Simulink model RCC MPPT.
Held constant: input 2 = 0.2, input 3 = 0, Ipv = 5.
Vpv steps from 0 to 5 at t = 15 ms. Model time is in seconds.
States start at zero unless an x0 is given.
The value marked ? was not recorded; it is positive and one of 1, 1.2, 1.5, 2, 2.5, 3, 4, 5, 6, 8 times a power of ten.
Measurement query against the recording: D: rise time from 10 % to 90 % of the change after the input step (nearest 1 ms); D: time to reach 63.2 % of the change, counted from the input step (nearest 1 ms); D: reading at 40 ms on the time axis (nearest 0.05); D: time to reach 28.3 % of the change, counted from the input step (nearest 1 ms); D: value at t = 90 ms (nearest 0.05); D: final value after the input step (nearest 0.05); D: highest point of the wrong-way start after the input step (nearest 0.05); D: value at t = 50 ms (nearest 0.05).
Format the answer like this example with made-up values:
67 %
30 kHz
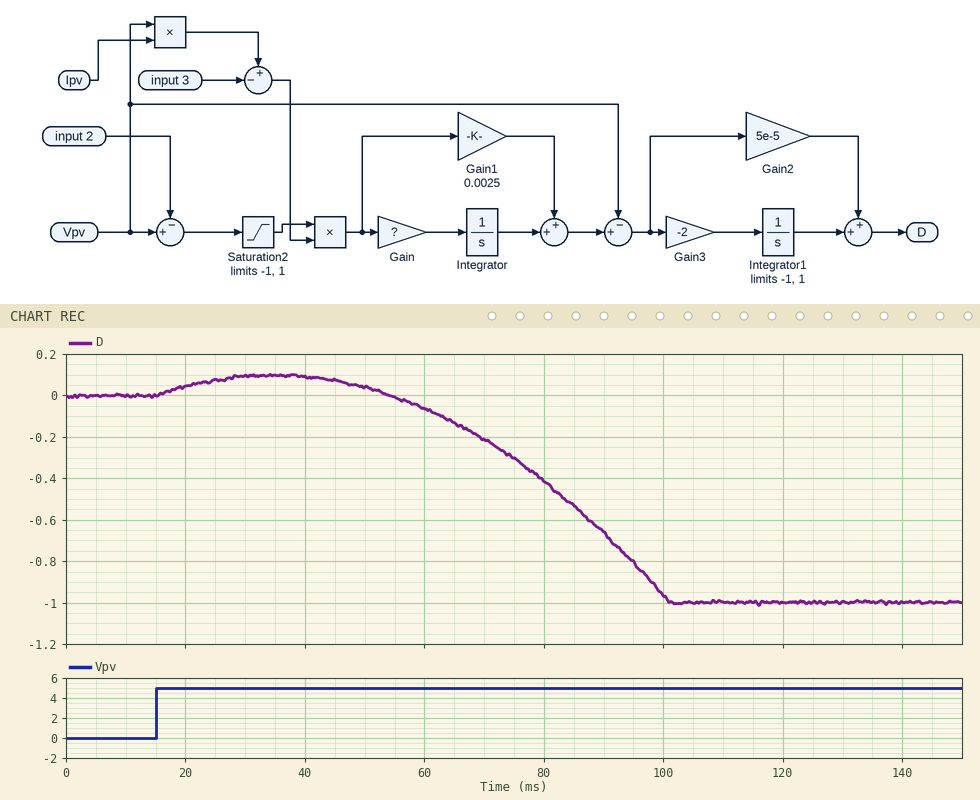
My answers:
35 ms
74 ms
0.10
59 ms
-0.65
-1.00
0.10
0.05
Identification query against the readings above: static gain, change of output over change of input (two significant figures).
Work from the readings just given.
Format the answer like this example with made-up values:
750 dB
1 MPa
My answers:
-0.20
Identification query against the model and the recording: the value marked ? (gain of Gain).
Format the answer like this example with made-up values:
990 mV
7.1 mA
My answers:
10
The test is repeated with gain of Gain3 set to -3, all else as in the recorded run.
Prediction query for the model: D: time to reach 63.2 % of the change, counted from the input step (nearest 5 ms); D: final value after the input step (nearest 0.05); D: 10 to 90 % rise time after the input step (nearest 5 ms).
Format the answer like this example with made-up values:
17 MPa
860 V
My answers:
65 ms
-1.00
25 ms
